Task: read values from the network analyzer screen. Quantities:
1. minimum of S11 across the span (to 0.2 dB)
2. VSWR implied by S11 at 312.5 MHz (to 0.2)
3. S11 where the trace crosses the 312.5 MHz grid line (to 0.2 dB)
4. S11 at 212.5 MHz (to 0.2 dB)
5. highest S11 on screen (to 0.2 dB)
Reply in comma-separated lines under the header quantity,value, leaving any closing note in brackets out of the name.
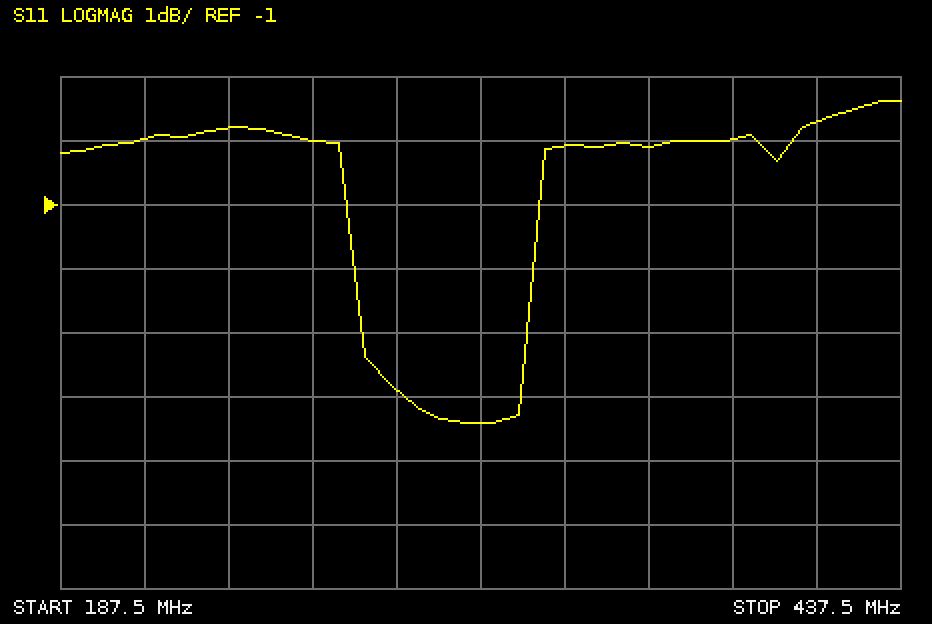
quantity,value
minimum of S11 across the span,-4.4 dB
VSWR implied by S11 at 312.5 MHz,4.0
S11 where the trace crosses the 312.5 MHz grid line,-4.4 dB
S11 at 212.5 MHz,0.0 dB
highest S11 on screen,0.6 dB
